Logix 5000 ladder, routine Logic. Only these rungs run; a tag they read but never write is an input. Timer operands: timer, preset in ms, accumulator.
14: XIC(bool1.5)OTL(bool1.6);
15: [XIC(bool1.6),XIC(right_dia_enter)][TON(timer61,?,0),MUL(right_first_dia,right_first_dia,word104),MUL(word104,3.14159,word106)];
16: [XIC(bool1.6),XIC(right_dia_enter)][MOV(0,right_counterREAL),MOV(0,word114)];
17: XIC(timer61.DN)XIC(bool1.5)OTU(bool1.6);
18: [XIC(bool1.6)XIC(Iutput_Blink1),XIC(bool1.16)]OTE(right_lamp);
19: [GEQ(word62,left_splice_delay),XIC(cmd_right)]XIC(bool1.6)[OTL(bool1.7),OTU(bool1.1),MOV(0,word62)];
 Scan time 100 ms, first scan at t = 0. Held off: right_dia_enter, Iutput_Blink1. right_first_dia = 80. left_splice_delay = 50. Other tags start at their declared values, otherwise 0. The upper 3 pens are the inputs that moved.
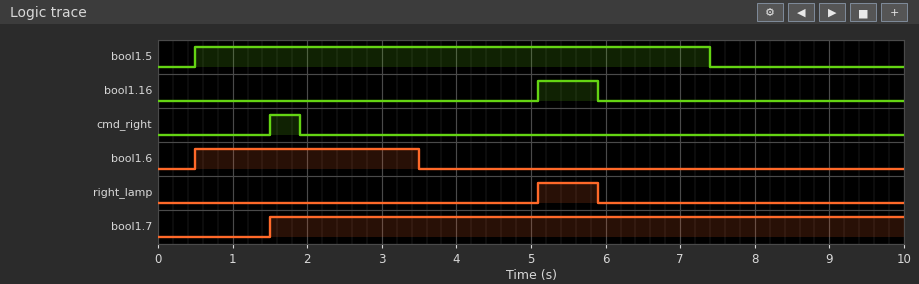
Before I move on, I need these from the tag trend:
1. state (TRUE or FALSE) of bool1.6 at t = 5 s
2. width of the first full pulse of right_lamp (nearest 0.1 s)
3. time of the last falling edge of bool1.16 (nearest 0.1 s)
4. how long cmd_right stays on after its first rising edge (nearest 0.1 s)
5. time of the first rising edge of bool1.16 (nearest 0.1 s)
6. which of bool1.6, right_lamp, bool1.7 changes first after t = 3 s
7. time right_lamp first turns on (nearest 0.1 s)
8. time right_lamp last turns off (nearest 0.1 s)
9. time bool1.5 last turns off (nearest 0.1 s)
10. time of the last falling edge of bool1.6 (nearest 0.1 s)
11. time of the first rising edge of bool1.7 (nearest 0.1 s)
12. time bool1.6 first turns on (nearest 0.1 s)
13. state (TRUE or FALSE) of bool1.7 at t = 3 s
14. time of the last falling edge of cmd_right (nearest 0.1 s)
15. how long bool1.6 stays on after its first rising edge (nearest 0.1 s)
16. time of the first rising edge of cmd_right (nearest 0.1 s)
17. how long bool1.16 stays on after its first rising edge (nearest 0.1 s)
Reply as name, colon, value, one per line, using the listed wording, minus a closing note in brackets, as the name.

state (TRUE or FALSE) of bool1.6 at t = 5 s: FALSE
width of the first full pulse of right_lamp: 0.8 s
time of the last falling edge of bool1.16: 5.9 s
how long cmd_right stays on after its first rising edge: 0.4 s
time of the first rising edge of bool1.16: 5.1 s
which of bool1.6, right_lamp, bool1.7 changes first after t = 3 s: bool1.6
time right_lamp first turns on: 5.1 s
time right_lamp last turns off: 5.9 s
time bool1.5 last turns off: 7.4 s
time of the last falling edge of bool1.6: 3.5 s
time of the first rising edge of bool1.7: 1.5 s
time bool1.6 first turns on: 0.5 s
state (TRUE or FALSE) of bool1.7 at t = 3 s: TRUE
time of the last falling edge of cmd_right: 1.9 s
how long bool1.6 stays on after its first rising edge: 3.0 s
time of the first rising edge of cmd_right: 1.5 s
how long bool1.16 stays on after its first rising edge: 0.8 s
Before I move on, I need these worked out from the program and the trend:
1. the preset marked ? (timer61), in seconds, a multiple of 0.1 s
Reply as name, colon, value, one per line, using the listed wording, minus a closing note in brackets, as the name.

the preset marked ? (timer61), in seconds, a multiple of 0.1 s: 3.0 s
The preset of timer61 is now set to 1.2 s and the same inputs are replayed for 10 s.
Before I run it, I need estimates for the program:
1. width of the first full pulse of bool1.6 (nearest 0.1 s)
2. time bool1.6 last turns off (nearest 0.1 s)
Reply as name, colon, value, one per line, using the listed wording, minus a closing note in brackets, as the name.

width of the first full pulse of bool1.6: 1.2 s
time bool1.6 last turns off: 1.7 s
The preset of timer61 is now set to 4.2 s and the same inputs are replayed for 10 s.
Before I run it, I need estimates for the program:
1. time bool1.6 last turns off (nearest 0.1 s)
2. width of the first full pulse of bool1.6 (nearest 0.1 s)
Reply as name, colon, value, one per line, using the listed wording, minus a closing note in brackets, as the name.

time bool1.6 last turns off: 4.7 s
width of the first full pulse of bool1.6: 4.2 s
